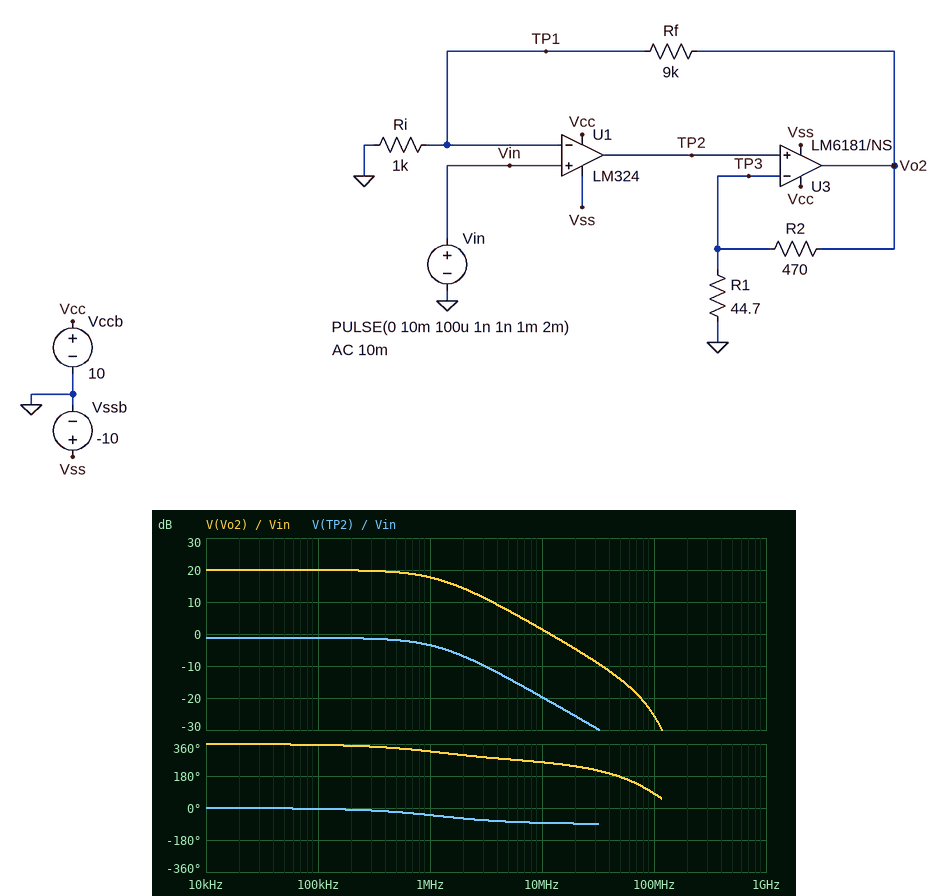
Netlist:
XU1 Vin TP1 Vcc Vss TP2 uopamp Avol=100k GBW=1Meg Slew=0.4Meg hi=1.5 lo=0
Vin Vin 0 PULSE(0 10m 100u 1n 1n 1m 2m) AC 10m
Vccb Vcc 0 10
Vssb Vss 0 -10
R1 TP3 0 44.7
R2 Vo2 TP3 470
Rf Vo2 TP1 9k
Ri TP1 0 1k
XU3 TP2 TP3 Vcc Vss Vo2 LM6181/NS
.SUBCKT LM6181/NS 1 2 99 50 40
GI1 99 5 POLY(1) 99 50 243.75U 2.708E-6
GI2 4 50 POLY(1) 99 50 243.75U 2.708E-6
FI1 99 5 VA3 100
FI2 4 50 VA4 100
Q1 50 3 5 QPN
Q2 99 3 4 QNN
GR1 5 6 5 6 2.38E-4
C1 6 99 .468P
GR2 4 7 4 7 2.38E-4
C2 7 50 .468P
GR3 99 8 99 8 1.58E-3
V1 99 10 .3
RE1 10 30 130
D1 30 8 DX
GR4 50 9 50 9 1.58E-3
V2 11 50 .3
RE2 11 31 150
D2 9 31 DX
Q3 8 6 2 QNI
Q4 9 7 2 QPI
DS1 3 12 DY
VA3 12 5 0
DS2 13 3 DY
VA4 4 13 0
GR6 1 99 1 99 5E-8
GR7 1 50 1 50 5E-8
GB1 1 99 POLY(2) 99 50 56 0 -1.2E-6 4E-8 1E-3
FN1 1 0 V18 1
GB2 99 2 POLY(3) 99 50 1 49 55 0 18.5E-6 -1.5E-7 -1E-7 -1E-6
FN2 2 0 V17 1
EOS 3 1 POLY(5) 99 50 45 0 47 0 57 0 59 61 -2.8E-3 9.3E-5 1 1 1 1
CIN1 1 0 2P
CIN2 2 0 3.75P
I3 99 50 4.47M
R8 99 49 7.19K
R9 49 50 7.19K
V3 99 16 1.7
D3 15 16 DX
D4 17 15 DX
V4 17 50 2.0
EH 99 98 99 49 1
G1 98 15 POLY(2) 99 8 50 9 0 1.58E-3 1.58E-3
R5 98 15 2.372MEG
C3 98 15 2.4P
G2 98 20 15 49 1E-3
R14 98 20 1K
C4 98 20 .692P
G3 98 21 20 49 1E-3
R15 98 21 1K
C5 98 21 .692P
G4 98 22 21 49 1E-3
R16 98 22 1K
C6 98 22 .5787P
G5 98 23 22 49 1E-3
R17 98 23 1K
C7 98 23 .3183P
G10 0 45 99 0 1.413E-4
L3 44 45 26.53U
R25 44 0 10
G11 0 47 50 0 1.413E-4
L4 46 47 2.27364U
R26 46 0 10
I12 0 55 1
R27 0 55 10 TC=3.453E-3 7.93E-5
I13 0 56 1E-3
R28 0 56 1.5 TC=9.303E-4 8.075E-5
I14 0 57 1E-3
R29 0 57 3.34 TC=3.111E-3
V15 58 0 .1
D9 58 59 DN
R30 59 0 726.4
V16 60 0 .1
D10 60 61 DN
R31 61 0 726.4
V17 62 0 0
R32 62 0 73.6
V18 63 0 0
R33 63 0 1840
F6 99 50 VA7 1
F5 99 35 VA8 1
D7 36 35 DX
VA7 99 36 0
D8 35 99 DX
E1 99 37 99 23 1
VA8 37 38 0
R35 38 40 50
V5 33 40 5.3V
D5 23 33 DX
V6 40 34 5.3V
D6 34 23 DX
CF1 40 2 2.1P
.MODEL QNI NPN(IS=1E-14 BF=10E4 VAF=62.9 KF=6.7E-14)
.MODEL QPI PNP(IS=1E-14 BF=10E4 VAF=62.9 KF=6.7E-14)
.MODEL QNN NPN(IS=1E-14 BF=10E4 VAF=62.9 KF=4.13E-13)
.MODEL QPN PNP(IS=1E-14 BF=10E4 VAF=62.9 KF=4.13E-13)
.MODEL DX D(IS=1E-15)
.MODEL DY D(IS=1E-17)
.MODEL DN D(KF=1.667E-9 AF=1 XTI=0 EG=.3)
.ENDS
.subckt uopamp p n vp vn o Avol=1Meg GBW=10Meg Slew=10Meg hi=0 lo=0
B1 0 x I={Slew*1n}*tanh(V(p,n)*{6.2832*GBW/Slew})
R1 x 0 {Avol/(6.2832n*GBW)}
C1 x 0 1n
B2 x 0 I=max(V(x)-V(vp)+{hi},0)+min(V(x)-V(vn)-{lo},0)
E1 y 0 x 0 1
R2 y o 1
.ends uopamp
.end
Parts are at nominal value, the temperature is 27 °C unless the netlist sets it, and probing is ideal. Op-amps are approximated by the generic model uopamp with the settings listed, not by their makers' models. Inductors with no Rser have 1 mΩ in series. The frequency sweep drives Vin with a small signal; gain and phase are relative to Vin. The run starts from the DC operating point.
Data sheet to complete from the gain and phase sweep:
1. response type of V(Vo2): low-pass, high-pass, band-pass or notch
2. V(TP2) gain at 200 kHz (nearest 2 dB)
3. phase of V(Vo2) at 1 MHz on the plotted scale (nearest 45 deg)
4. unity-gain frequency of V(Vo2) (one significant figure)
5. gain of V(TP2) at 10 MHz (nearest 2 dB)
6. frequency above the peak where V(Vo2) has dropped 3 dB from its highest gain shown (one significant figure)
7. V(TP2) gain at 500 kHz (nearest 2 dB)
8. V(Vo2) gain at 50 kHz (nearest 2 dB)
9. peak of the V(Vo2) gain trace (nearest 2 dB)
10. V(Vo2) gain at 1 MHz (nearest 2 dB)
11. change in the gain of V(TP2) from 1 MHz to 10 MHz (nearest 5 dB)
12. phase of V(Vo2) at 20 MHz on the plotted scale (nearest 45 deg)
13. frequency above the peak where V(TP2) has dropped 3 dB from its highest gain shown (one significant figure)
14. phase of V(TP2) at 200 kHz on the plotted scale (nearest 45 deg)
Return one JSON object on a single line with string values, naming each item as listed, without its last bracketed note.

{"response type of V(Vo2): low-pass, high-pass, band-pass or notch": "low-pass", "V(TP2) gain at 200 kHz": "-2 dB", "phase of V(Vo2) at 1 MHz on the plotted scale": "315 deg", "unity-gain frequency of V(Vo2)": "10 MHz", "gain of V(TP2) at 10 MHz": "-20 dB", "frequency above the peak where V(Vo2) has dropped 3 dB from its highest gain shown": "1 MHz", "V(TP2) gain at 500 kHz": "-2 dB", "V(Vo2) gain at 50 kHz": "20 dB", "peak of the V(Vo2) gain trace": "20 dB", "V(Vo2) gain at 1 MHz": "18 dB", "change in the gain of V(TP2) from 1 MHz to 10 MHz": "-15 dB", "phase of V(Vo2) at 20 MHz on the plotted scale": "225 deg", "frequency above the peak where V(TP2) has dropped 3 dB from its highest gain shown": "1 MHz", "phase of V(TP2) at 200 kHz on the plotted scale": "0 deg"}
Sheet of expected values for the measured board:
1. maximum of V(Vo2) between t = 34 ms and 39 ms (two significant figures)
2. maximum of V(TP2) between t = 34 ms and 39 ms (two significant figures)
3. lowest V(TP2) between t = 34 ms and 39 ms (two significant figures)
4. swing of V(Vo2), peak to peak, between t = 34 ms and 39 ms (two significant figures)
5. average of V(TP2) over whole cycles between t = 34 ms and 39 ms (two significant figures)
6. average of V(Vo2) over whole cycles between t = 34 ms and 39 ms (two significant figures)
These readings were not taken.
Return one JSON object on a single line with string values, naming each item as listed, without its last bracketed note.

{"maximum of V(Vo2) between t = 34 ms and 39 ms": "100 mV", "maximum of V(TP2) between t = 34 ms and 39 ms": "6.5 mV", "lowest V(TP2) between t = 34 ms and 39 ms": "-2.2 mV", "swing of V(Vo2), peak to peak, between t = 34 ms and 39 ms": "100 mV", "average of V(TP2) over whole cycles between t = 34 ms and 39 ms": "2.2 mV", "average of V(Vo2) over whole cycles between t = 34 ms and 39 ms": "50 mV"}
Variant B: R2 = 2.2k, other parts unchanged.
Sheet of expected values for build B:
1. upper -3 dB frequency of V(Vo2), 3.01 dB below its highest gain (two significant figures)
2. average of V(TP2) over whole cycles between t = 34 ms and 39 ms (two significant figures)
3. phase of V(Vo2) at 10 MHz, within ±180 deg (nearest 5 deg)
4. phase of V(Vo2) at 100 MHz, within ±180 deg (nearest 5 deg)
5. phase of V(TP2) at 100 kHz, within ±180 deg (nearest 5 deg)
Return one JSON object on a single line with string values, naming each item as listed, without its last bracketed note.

{"upper -3 dB frequency of V(Vo2), 3.01 dB below its highest gain": "7.9 MHz", "average of V(TP2) over whole cycles between t = 34 ms and 39 ms": "-1.2 mV", "phase of V(Vo2) at 10 MHz, within ±180 deg": "-125 deg", "phase of V(Vo2) at 100 MHz, within ±180 deg": "70 deg", "phase of V(TP2) at 100 kHz, within ±180 deg": "0 deg"}
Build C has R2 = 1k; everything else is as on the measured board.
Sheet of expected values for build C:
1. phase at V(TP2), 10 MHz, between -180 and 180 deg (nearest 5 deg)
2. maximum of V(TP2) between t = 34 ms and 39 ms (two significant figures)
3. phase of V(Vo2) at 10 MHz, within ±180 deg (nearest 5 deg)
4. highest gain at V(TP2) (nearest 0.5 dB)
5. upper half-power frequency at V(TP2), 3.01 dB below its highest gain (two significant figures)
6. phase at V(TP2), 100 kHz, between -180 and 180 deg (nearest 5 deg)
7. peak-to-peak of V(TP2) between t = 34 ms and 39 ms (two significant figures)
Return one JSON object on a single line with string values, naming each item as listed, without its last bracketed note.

{"phase at V(TP2), 10 MHz, between -180 and 180 deg": "-80 deg", "maximum of V(TP2) between t = 34 ms and 39 ms": "2.1 mV", "phase of V(Vo2) at 10 MHz, within ±180 deg": "-110 deg", "highest gain at V(TP2)": "-7.5 dB", "upper half-power frequency at V(TP2), 3.01 dB below its highest gain": "2.7 MHz", "phase at V(TP2), 100 kHz, between -180 and 180 deg": "0 deg", "peak-to-peak of V(TP2) between t = 34 ms and 39 ms": "4.3 mV"}
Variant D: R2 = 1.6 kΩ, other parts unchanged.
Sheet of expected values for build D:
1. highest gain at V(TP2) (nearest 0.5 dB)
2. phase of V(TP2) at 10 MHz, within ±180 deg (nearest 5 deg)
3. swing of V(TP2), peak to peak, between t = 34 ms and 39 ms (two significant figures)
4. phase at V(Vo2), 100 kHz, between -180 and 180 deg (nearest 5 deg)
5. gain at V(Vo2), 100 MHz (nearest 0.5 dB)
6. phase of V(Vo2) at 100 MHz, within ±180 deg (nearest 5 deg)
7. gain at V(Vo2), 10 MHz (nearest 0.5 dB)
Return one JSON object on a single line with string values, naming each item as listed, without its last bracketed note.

{"highest gain at V(TP2)": "-11.5 dB", "phase of V(TP2) at 10 MHz, within ±180 deg": "-75 deg", "swing of V(TP2), peak to peak, between t = 34 ms and 39 ms": "2.7 mV", "phase at V(Vo2), 100 kHz, between -180 and 180 deg": "0 deg", "gain at V(Vo2), 100 MHz": "-28.5 dB", "phase of V(Vo2) at 100 MHz, within ±180 deg": "70 deg", "gain at V(Vo2), 10 MHz": "11.5 dB"}
